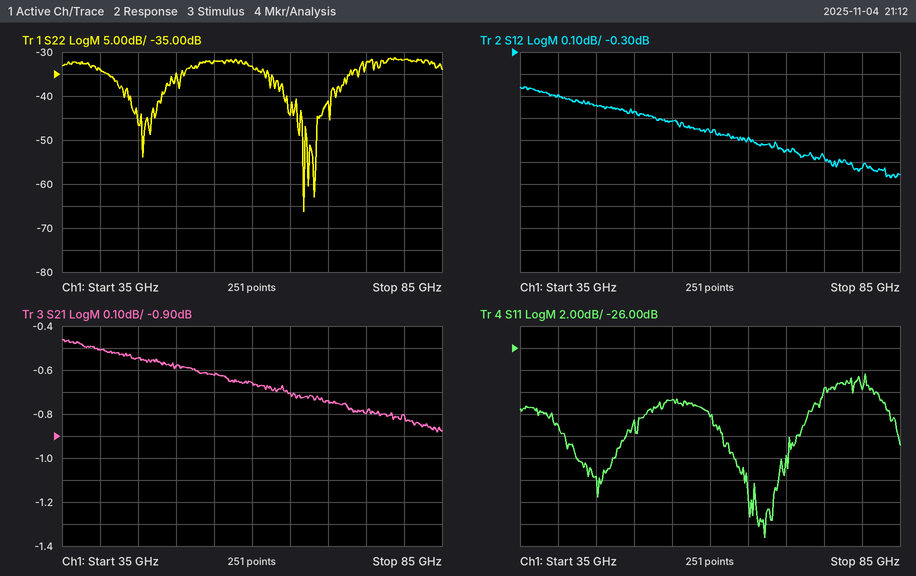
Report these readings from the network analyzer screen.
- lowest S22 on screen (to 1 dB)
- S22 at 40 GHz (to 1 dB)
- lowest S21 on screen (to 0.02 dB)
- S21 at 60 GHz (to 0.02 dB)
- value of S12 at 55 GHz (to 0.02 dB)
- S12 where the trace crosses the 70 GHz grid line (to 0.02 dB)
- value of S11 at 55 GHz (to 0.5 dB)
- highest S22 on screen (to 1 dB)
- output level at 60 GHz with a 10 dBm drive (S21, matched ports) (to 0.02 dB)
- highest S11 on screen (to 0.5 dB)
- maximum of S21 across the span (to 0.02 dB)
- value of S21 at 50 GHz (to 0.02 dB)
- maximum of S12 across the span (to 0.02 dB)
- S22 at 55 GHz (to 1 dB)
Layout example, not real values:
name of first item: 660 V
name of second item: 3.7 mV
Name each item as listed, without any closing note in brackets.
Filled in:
lowest S22 on screen: -66 dB
S22 at 40 GHz: -34 dB
lowest S21 on screen: -0.88 dB
S21 at 60 GHz: -0.66 dB
value of S12 at 55 GHz: -0.62 dB
S12 where the trace crosses the 70 GHz grid line: -0.74 dB
value of S11 at 55 GHz: -30.5 dB
highest S22 on screen: -31 dB
output level at 60 GHz with a 10 dBm drive (S21, matched ports): 9.34 dBm
highest S11 on screen: -28.5 dB
maximum of S21 across the span: -0.46 dB
value of S21 at 50 GHz: -0.58 dB
maximum of S12 across the span: -0.46 dB
S22 at 55 GHz: -32 dB
